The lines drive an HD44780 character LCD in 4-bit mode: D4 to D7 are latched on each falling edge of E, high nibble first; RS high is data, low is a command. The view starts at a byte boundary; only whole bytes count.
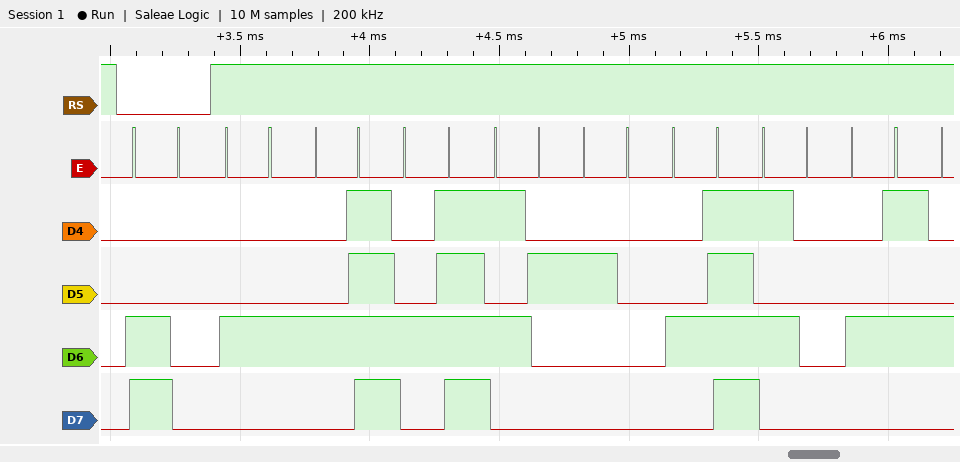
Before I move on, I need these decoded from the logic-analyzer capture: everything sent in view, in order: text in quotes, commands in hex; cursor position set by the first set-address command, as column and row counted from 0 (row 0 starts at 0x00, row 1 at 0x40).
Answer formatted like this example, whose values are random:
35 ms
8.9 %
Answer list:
0xC0 "DOOR OPE"
column 0, row 1
